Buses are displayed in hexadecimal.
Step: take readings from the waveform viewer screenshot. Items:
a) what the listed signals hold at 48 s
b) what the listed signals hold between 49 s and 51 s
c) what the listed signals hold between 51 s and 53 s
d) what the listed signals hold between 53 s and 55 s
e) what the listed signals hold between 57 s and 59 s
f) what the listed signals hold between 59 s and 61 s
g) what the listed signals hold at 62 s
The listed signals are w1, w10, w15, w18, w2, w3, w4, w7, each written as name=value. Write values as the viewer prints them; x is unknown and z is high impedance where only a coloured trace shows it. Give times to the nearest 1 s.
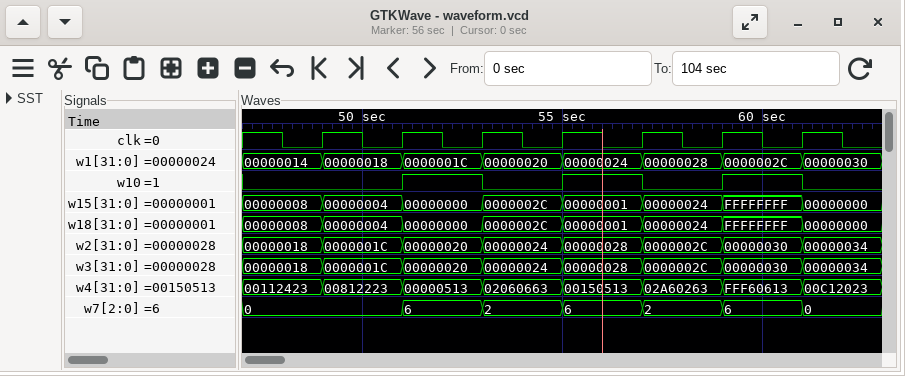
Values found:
w1=00000014, w10=0, w15=00000008, w18=00000008, w2=00000018, w3=00000018, w4=00112423, w7=0
w1=00000018, w10=0, w15=00000004, w18=00000004, w2=0000001C, w3=0000001C, w4=00812223, w7=0
w1=0000001C, w10=1, w15=00000000, w18=00000000, w2=00000020, w3=00000020, w4=00000513, w7=6
w1=00000020, w10=0, w15=0000002C, w18=0000002C, w2=00000024, w3=00000024, w4=02060663, w7=2
w1=00000028, w10=0, w15=00000024, w18=00000024, w2=0000002C, w3=0000002C, w4=02A60263, w7=2
w1=0000002C, w10=1, w15=FFFFFFFF, w18=FFFFFFFF, w2=00000030, w3=00000030, w4=FFF60613, w7=6
w1=00000030, w10=0, w15=00000000, w18=00000000, w2=00000034, w3=00000034, w4=00C12023, w7=0
